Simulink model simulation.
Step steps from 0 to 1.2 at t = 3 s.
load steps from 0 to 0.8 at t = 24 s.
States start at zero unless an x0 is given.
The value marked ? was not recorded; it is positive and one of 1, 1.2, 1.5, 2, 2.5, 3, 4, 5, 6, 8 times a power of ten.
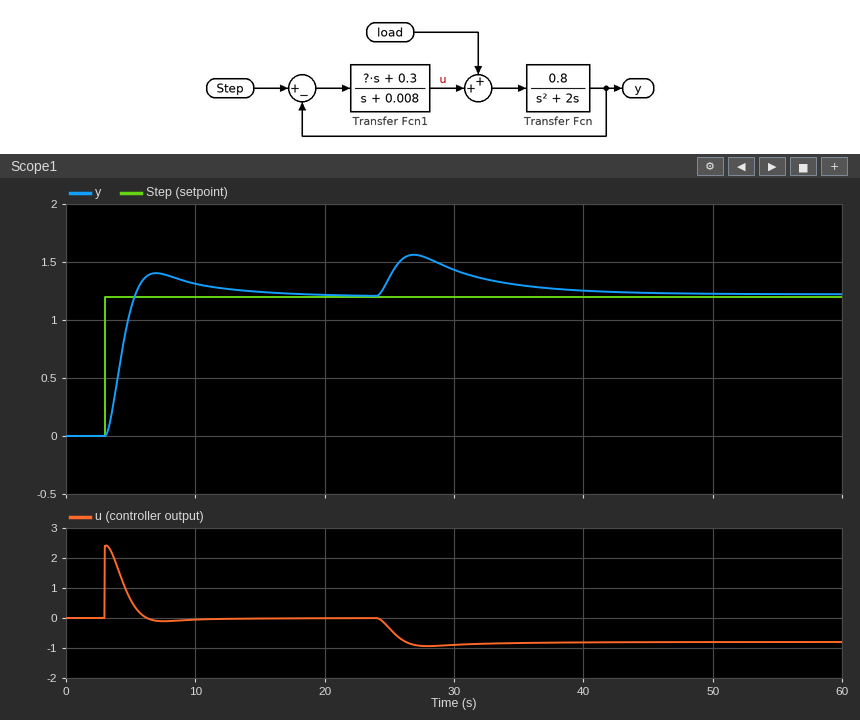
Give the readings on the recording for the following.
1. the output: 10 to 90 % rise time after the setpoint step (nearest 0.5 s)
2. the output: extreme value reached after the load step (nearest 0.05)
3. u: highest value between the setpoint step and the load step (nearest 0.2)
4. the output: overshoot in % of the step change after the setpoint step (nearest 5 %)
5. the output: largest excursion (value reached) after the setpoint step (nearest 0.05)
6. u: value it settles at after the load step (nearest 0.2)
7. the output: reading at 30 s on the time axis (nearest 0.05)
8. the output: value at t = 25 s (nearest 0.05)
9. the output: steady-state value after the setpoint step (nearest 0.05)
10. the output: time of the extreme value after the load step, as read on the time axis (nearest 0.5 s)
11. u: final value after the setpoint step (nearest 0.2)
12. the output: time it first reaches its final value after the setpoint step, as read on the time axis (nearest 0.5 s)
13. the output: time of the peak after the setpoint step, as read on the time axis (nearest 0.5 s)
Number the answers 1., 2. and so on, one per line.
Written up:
1. 1.5 s
2. 1.55
3. 2.4
4. 15 %
5. 1.40
6. -0.8
7. 1.45
8. 1.35
9. 1.20
10. 27.0 s
11. 0.0
12. 5.5 s
13. 7.0 s
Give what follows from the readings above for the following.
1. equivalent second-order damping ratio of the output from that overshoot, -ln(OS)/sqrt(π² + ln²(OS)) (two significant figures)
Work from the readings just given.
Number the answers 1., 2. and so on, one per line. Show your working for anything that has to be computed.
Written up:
1. ln(0.15) = -1.897; 1.897 / sqrt(9.870 + 3.599) = 0.52
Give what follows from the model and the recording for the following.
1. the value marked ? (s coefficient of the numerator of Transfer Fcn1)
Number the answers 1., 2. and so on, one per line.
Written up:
1. 2
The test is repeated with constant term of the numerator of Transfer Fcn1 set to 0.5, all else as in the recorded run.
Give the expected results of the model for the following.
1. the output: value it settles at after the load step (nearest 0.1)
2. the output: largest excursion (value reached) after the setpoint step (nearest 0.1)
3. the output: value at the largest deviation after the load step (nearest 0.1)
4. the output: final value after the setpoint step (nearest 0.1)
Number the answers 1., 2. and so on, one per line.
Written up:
1. 1.2
2. 1.5
3. 1.5
4. 1.2
